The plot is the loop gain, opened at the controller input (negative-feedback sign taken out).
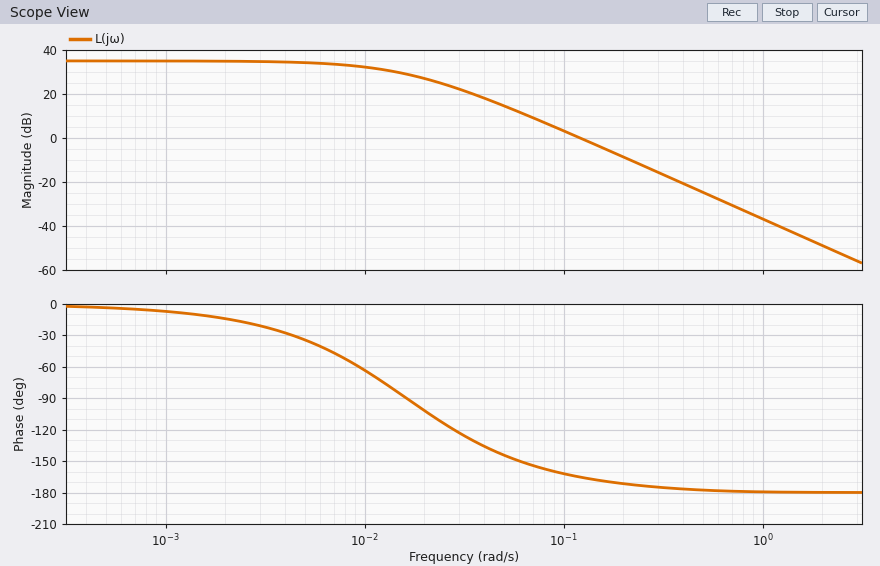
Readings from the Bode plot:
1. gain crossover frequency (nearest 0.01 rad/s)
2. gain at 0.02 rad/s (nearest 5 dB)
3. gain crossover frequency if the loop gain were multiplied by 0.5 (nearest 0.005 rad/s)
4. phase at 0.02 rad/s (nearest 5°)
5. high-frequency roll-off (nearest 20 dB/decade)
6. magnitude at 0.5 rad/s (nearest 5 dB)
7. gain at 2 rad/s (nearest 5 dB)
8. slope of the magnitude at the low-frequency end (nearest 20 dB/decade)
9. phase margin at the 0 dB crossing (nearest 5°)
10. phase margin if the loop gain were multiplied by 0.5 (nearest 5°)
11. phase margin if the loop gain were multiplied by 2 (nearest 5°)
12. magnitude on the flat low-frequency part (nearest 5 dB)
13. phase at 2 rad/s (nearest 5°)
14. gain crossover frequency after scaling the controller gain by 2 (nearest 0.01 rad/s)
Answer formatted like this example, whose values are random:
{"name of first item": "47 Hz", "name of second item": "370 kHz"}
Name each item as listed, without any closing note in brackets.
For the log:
{"gain crossover frequency": "0.12 rad/s", "gain at 0.02 rad/s": "25 dB", "gain crossover frequency if the loop gain were multiplied by 0.5": "0.085 rad/s", "phase at 0.02 rad/s": "-100°", "high-frequency roll-off": "-40 dB/decade", "magnitude at 0.5 rad/s": "-25 dB", "gain at 2 rad/s": "-50 dB", "slope of the magnitude at the low-frequency end": "0 dB/decade", "phase margin at the 0 dB crossing": "15°", "phase margin if the loop gain were multiplied by 0.5": "20°", "phase margin if the loop gain were multiplied by 2": "10°", "magnitude on the flat low-frequency part": "35 dB", "phase at 2 rad/s": "-180°", "gain crossover frequency after scaling the controller gain by 2": "0.17 rad/s"}
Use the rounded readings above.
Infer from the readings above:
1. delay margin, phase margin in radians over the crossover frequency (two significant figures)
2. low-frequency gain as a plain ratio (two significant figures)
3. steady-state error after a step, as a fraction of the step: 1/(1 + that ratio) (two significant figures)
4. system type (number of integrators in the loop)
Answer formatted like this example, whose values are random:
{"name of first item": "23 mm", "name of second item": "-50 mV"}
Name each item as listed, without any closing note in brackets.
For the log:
{"delay margin, phase margin in radians over the crossover frequency": "2.2 s", "low-frequency gain as a plain ratio": "56", "steady-state error after a step, as a fraction of the step: 1/(1 + that ratio)": "0.018", "system type": "0"}
